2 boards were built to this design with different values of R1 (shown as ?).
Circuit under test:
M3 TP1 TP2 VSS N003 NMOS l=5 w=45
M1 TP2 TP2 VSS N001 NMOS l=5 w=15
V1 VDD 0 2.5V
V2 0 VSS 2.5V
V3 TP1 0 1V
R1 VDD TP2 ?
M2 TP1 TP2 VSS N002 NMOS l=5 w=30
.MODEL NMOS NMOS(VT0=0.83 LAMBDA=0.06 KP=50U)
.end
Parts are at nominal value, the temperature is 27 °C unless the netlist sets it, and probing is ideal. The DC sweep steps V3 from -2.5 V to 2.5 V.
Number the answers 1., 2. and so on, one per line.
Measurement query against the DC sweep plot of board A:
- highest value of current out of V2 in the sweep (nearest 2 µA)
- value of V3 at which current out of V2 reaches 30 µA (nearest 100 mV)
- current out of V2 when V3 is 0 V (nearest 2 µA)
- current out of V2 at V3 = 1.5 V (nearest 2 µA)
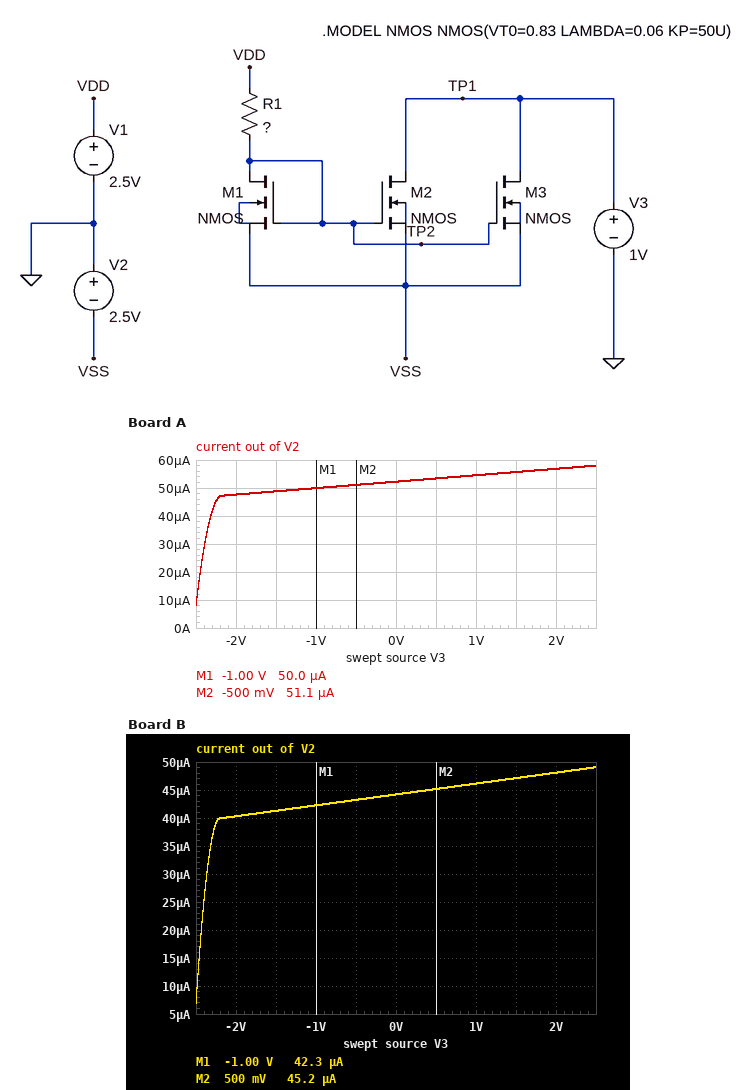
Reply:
1. 58 µA
2. -2.4 V
3. 52 µA
4. 56 µA
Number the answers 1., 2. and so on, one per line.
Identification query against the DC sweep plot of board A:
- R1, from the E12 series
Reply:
1. 470 kΩ
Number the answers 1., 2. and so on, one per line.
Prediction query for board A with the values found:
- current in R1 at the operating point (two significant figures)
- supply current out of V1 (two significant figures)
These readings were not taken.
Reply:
1. 8.2 µA
2. 8.2 µA
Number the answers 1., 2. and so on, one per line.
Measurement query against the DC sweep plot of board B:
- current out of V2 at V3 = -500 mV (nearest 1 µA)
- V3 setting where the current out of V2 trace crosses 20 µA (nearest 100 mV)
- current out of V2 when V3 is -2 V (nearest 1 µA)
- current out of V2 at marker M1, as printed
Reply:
1. 43 µA
2. -2.4 V
3. 40 µA
4. 42.3 µA
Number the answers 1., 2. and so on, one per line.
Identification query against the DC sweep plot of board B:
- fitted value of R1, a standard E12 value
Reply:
1. 560 kΩ
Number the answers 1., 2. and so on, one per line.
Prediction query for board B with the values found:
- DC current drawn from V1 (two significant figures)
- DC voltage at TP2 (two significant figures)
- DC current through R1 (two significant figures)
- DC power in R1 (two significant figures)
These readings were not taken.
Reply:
1. 6.9 µA
2. -1.4 V
3. 6.9 µA
4. 27 µW
